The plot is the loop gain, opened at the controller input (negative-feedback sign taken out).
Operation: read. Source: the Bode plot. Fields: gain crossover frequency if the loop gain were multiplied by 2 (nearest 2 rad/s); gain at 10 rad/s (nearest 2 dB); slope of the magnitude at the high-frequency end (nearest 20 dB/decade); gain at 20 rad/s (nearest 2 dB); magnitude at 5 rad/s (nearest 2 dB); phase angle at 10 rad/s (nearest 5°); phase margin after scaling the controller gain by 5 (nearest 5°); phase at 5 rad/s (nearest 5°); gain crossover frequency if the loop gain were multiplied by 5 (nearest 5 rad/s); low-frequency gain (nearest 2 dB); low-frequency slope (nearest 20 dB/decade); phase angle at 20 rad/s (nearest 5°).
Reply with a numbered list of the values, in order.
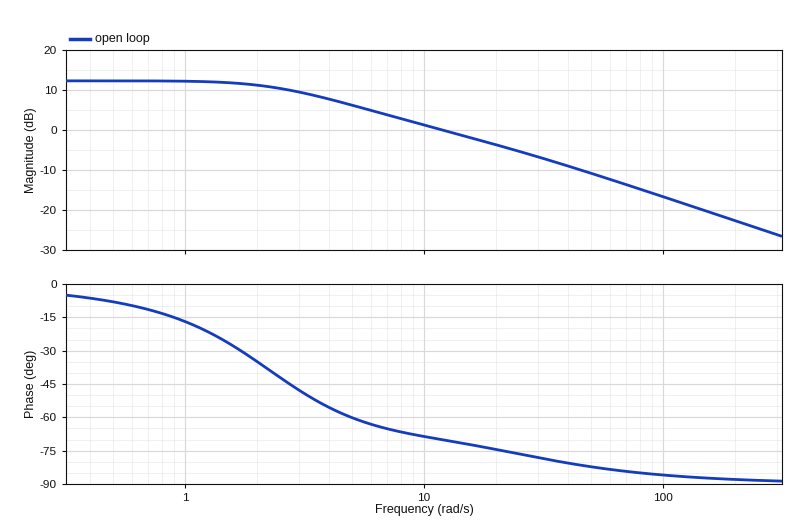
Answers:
1. 28 rad/s
2. 2 dB
3. -20 dB/decade
4. -4 dB
5. 6 dB
6. -70°
7. 95°
8. -60°
9. 75 rad/s
10. 12 dB
11. 0 dB/decade
12. -75°
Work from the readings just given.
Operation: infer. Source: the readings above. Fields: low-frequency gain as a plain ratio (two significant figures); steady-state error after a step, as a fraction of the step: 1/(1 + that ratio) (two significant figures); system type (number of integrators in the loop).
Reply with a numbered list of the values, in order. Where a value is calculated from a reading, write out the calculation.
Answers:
1. 10^(12 / 20) = 4.0
2. 1 / (1 + 4) = 0.20
3. 0
